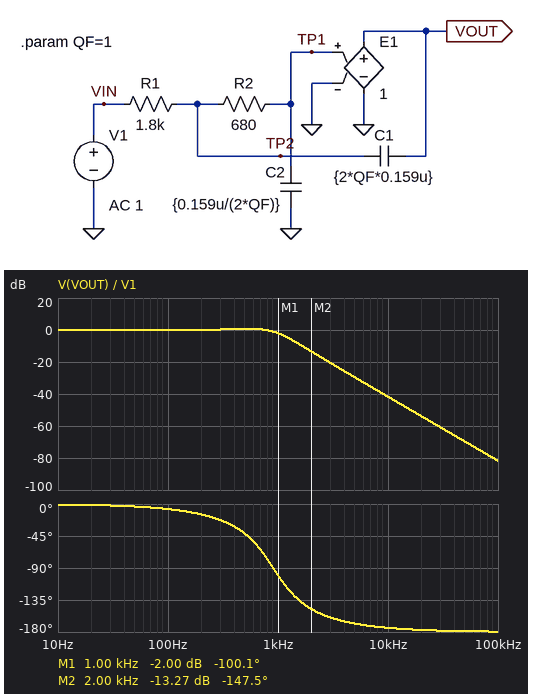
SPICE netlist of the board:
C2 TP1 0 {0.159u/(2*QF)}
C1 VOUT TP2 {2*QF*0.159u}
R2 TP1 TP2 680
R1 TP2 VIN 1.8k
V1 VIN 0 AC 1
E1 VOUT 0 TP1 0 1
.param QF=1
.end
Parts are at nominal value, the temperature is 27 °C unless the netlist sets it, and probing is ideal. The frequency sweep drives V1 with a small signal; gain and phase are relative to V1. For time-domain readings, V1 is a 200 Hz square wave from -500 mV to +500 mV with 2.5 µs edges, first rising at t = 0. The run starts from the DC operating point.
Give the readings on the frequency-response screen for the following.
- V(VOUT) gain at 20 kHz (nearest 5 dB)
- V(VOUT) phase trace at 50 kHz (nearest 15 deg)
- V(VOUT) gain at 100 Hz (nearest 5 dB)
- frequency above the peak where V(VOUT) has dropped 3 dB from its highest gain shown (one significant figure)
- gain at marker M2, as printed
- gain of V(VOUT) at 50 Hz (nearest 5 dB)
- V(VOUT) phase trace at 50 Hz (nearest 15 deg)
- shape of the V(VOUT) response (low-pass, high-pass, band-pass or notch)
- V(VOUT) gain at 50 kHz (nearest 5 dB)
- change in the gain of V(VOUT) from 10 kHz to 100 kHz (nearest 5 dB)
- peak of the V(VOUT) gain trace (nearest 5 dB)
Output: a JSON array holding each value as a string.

["-55 dB", "-180 deg", "0 dB", "1 kHz", "-13.27 dB", "0 dB", "0 deg", "low-pass", "-70 dB", "-40 dB", "0 dB"]
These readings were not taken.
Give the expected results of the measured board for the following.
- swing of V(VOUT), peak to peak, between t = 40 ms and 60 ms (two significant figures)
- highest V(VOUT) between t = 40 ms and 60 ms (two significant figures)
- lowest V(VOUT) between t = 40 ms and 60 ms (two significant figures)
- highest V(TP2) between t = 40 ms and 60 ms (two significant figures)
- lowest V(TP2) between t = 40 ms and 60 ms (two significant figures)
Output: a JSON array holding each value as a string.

["1.2 V", "620 mV", "-620 mV", "630 mV", "-630 mV"]
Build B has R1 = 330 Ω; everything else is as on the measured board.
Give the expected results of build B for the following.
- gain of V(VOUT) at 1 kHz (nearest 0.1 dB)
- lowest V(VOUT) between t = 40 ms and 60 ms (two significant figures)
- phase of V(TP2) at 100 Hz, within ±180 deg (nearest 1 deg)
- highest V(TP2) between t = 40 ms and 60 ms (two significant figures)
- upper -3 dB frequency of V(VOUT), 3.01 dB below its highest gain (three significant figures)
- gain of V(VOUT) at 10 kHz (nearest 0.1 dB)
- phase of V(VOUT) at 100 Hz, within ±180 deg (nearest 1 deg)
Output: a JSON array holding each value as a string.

["0.7 dB", "-640 mV", "-1 deg", "700 mV", "2.44 kHz", "-26.8 dB", "-3 deg"]
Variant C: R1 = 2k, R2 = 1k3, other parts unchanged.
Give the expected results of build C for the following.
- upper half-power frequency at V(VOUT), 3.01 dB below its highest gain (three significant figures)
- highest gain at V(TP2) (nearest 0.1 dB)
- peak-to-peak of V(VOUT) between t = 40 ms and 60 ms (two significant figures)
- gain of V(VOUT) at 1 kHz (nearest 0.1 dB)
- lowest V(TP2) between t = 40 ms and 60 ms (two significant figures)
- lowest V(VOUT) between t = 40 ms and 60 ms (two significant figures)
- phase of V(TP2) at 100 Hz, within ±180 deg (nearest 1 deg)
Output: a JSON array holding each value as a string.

["723 Hz", "1.5 dB", "1.3 V", "-7.2 dB", "-670 mV", "-650 mV", "-6 deg"]
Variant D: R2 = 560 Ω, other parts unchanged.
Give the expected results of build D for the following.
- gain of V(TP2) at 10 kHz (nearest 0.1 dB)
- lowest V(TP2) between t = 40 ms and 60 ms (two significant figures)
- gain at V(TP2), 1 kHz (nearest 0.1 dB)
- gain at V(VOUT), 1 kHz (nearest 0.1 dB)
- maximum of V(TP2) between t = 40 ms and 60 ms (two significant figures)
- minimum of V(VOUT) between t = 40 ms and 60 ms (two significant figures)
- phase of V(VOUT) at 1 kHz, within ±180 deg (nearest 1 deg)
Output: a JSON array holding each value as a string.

["-30.6 dB", "-610 mV", "-1.1 dB", "-1.4 dB", "610 mV", "-600 mV", "-90 deg"]
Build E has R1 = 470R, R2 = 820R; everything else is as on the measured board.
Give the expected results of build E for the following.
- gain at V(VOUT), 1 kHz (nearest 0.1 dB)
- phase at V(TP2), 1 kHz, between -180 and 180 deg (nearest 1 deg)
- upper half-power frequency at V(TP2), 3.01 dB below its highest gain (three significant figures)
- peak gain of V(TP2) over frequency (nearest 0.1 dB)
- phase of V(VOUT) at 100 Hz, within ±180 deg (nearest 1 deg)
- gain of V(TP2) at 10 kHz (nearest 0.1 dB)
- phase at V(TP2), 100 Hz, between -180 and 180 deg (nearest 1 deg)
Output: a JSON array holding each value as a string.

["1.0 dB", "-24 deg", "2.07 kHz", "1.9 dB", "-4 deg", "-19.1 dB", "-1 deg"]
